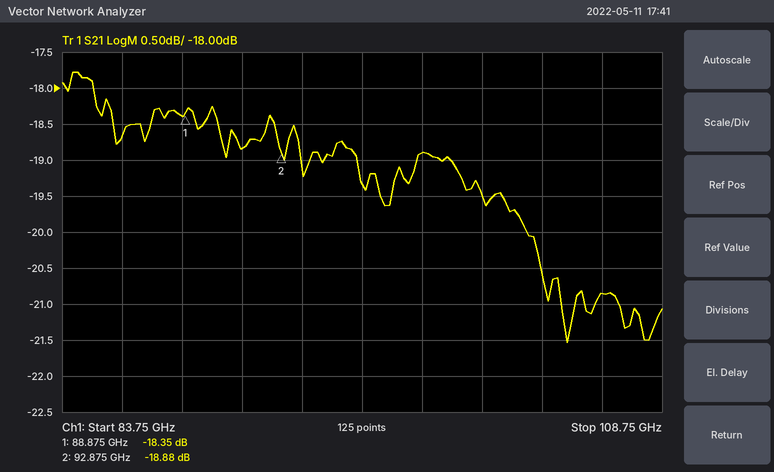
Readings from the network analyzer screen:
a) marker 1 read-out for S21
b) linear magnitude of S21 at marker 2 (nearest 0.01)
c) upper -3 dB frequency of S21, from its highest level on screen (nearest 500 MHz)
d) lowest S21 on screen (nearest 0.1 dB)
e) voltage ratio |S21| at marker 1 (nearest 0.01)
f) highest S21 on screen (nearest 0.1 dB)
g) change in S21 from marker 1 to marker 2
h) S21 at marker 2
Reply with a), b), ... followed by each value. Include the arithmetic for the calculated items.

a) -18.35 dB
b) 10^(-18.88/20) ≈ 0.11
c) 104.0 GHz
d) -21.5 dB
e) 10^(-18.35/20) ≈ 0.12
f) -17.8 dB
g) -18.88 − (-18.35) = -0.53 dB
h) -18.88 dB
